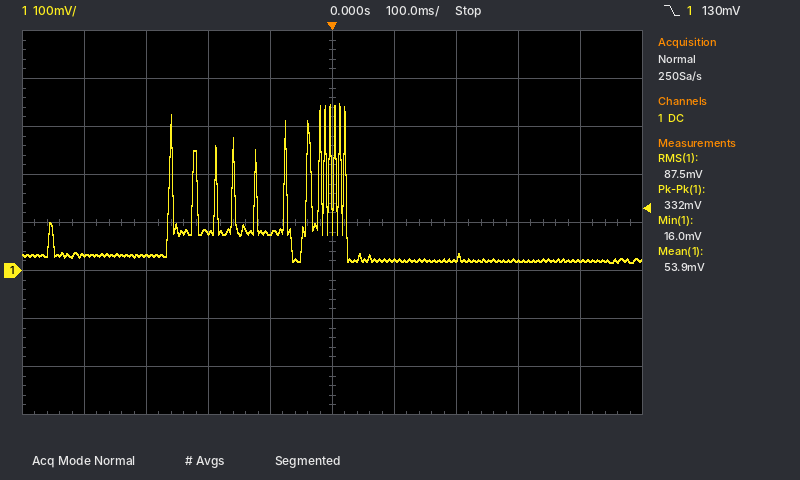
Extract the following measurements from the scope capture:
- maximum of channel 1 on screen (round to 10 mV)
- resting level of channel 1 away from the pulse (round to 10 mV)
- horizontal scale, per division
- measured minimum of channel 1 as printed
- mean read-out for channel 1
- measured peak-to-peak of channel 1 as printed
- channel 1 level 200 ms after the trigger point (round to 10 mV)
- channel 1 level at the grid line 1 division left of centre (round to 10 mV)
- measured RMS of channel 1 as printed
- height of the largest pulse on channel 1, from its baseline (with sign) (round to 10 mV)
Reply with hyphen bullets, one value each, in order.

- 350 mV
- 20 mV
- 100 ms
- 16.0 mV
- 53.9 mV
- 332 mV
- 30 mV
- 80 mV
- 87.5 mV
- +330 mV
